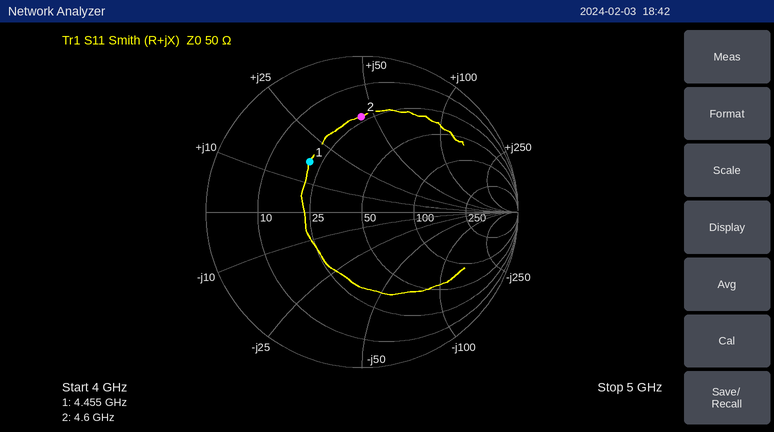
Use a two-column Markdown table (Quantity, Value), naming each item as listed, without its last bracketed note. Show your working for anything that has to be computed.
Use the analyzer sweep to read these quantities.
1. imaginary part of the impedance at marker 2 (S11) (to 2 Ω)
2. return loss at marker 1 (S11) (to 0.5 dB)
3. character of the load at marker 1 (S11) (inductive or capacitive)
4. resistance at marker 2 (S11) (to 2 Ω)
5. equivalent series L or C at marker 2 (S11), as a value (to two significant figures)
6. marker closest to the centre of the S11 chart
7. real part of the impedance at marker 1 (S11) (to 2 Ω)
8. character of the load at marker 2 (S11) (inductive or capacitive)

| Quantity | Value |
|---|---|
| imaginary part of the impedance at marker 2 (S11) | +44 Ω |
| return loss at marker 1 (S11) | 6.5 dB |
| character of the load at marker 1 (S11) | inductive |
| resistance at marker 2 (S11) | 22 Ω |
| equivalent series L or C at marker 2 (S11), as a value | L = 44 Ω/(2π × 4.6 GHz) ≈ 1.5 nH |
| marker closest to the centre of the S11 chart | marker 1 |
| real part of the impedance at marker 1 (S11) | 20 Ω |
| character of the load at marker 2 (S11) | inductive |
